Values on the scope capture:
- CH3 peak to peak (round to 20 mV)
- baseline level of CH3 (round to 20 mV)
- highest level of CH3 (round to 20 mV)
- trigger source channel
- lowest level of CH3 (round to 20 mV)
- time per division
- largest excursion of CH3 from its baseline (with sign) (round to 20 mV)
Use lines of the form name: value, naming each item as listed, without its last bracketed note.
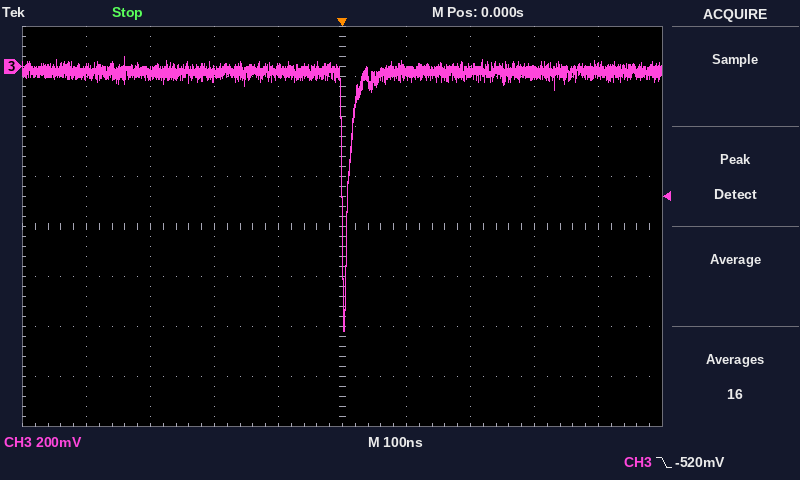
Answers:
CH3 peak to peak: 1.10 V
baseline level of CH3: -20 mV
highest level of CH3: 40 mV
trigger source channel: CH3
lowest level of CH3: -1.06 V
time per division: 100 ns
largest excursion of CH3 from its baseline (with sign): -1.04 V
